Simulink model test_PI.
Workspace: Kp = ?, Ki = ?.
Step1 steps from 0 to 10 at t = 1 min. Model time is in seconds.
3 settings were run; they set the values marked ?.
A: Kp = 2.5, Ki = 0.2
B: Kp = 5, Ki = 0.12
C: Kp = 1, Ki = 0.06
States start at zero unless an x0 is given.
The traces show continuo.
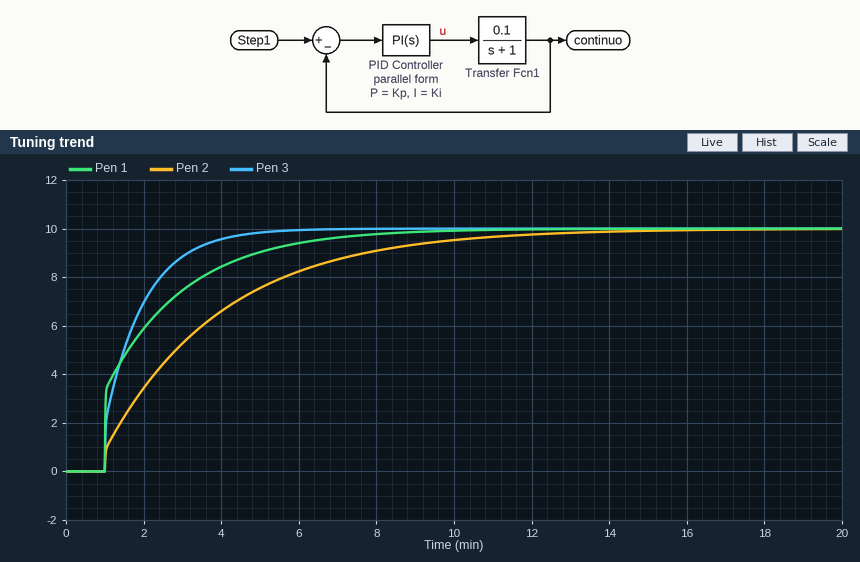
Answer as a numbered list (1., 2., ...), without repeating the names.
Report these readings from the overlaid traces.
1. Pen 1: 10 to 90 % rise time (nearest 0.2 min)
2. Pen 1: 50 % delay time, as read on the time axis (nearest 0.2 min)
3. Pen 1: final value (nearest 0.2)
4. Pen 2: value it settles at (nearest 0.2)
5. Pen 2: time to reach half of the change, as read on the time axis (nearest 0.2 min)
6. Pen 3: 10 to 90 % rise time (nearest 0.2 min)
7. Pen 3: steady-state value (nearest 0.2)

1. 4.0 min
2. 1.6 min
3. 10.0
4. 10.0
5. 2.8 min
6. 2.2 min
7. 10.0
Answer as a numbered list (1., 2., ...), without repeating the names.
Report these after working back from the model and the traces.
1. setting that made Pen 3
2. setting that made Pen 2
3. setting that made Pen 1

1. A
2. C
3. B
